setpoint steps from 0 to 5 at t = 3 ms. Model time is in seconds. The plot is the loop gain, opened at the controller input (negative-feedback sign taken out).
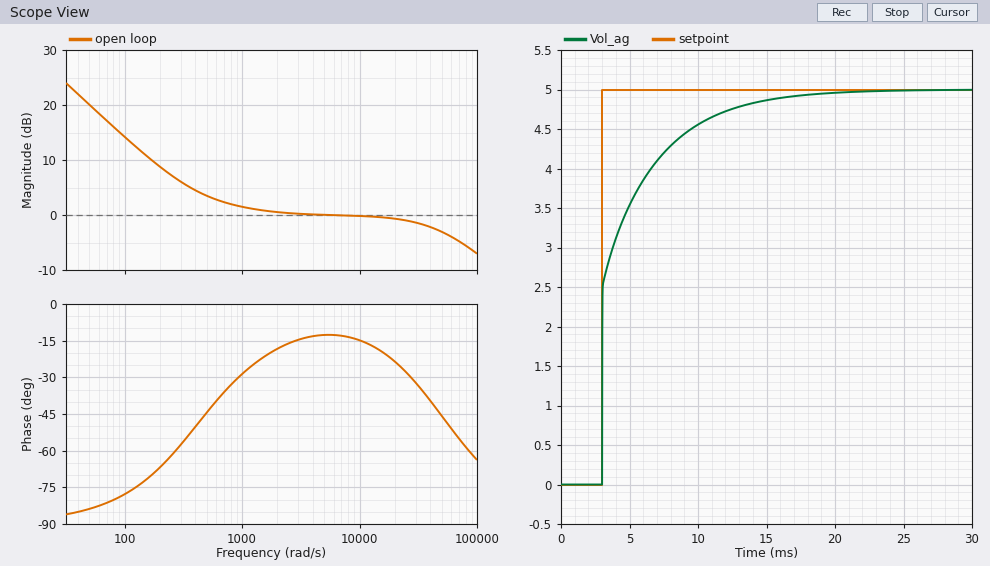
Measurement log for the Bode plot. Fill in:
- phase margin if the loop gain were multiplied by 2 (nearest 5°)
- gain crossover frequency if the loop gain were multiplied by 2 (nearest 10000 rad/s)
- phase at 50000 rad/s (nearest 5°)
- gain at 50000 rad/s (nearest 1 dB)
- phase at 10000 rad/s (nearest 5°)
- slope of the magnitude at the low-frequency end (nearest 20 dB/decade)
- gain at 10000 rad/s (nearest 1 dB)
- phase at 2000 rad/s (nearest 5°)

120°
90000 rad/s
-45°
-3 dB
-15°
-20 dB/decade
0 dB
-20°
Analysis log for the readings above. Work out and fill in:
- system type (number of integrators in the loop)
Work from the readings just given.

1
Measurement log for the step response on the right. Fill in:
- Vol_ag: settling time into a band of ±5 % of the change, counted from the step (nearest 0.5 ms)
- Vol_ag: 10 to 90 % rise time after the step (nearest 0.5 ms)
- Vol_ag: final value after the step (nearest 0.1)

9.5 ms
6.5 ms
5.0
